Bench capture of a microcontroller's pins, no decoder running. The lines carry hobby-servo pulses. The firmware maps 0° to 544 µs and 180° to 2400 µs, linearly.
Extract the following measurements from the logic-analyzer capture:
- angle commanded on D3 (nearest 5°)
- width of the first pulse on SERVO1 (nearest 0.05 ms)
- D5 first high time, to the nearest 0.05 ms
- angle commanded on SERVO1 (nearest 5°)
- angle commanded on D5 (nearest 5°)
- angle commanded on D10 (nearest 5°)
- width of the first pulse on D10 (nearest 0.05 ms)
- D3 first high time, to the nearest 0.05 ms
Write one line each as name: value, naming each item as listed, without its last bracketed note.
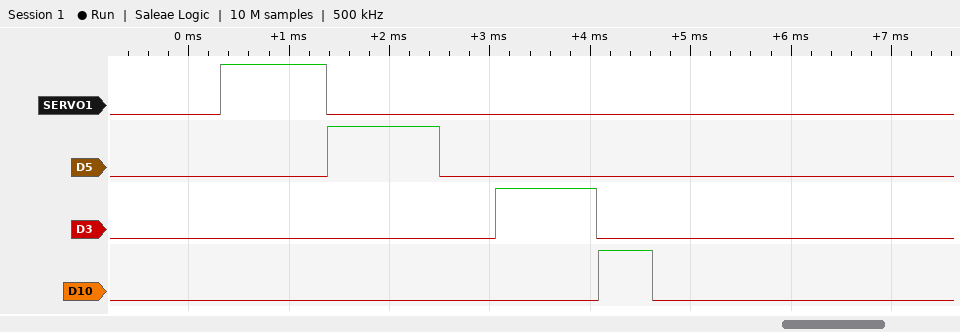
angle commanded on D3: 45°
width of the first pulse on SERVO1: 1.05 ms
D5 first high time, to the nearest 0.05 ms: 1.10 ms
angle commanded on SERVO1: 50°
angle commanded on D5: 55°
angle commanded on D10: 0°
width of the first pulse on D10: 0.55 ms
D3 first high time, to the nearest 0.05 ms: 1.00 ms
